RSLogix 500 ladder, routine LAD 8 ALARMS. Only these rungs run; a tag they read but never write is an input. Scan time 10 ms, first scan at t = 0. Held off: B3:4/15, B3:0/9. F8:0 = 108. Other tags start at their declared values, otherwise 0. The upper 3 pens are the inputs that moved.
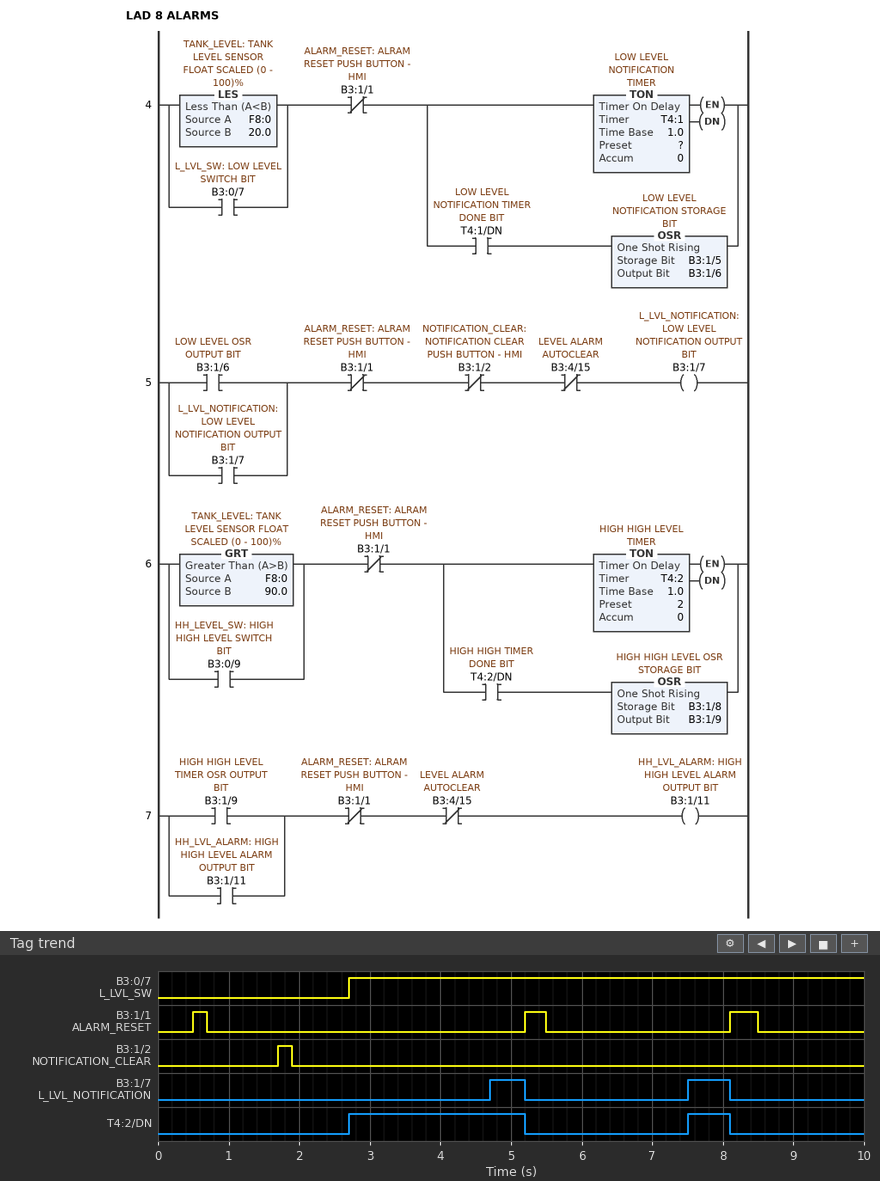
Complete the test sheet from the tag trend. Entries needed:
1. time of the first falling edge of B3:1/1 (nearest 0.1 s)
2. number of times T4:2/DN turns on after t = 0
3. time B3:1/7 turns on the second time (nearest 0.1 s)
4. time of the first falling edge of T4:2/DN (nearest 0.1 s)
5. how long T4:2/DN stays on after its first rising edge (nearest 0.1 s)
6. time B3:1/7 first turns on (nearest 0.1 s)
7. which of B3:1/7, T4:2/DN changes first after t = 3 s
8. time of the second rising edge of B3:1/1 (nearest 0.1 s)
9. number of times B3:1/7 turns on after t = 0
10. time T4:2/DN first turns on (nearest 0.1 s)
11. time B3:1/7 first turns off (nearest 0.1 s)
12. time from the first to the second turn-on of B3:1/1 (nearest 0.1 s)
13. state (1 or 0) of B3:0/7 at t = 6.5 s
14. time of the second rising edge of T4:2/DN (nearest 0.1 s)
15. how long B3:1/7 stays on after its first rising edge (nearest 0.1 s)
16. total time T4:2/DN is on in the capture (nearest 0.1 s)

0.7 s
2
7.5 s
5.2 s
2.5 s
4.7 s
B3:1/7
5.2 s
2
2.7 s
5.2 s
4.7 s
1
7.5 s
0.5 s
3.1 s
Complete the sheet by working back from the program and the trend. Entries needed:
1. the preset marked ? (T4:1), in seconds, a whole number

2 s
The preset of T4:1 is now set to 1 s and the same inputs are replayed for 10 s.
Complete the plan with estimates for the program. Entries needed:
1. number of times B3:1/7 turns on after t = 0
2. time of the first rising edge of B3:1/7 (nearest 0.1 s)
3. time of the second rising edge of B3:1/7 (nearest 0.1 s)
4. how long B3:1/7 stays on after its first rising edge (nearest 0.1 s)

3
3.7 s
6.5 s
1.5 s
